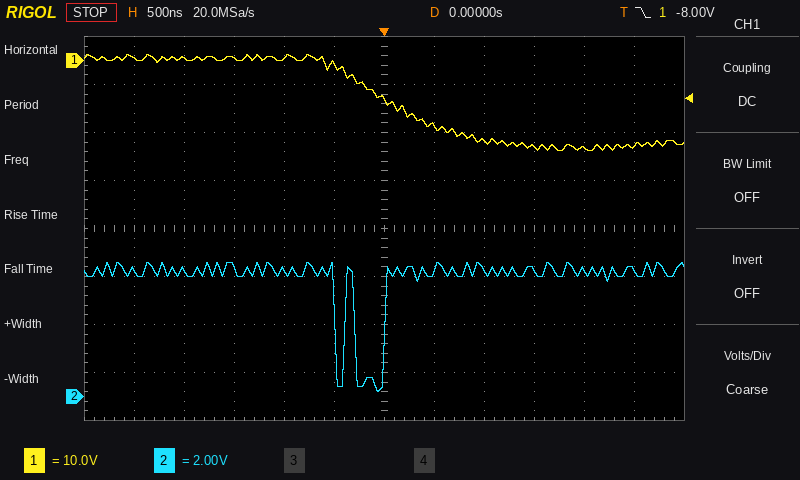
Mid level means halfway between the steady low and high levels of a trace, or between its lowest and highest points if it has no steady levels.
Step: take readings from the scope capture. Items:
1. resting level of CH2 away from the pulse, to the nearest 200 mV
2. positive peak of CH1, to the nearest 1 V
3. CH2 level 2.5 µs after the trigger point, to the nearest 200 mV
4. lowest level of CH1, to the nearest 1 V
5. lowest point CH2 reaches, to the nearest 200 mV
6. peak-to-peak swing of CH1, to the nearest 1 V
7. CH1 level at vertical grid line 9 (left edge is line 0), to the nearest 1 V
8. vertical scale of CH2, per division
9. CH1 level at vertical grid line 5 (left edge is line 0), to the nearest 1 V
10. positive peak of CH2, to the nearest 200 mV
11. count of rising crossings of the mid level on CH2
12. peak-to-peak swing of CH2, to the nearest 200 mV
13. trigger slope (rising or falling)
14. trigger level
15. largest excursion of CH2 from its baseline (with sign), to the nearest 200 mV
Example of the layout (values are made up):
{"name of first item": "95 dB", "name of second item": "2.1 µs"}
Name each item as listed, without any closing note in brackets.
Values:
{"resting level of CH2 away from the pulse, to the nearest 200 mV": "5.2 V", "positive peak of CH1, to the nearest 1 V": "1 V", "CH2 level 2.5 µs after the trigger point, to the nearest 200 mV": "5.2 V", "lowest level of CH1, to the nearest 1 V": "-19 V", "lowest point CH2 reaches, to the nearest 200 mV": "200 mV", "peak-to-peak swing of CH1, to the nearest 1 V": "20 V", "CH1 level at vertical grid line 9 (left edge is line 0), to the nearest 1 V": "-18 V", "vertical scale of CH2, per division": "2 V", "CH1 level at vertical grid line 5 (left edge is line 0), to the nearest 1 V": "-1 V", "positive peak of CH2, to the nearest 200 mV": "5.6 V", "count of rising crossings of the mid level on CH2": "2", "peak-to-peak swing of CH2, to the nearest 200 mV": "5.4 V", "trigger slope": "falling", "trigger level": "-8.00 V", "largest excursion of CH2 from its baseline (with sign), to the nearest 200 mV": "-5.0 V"}
